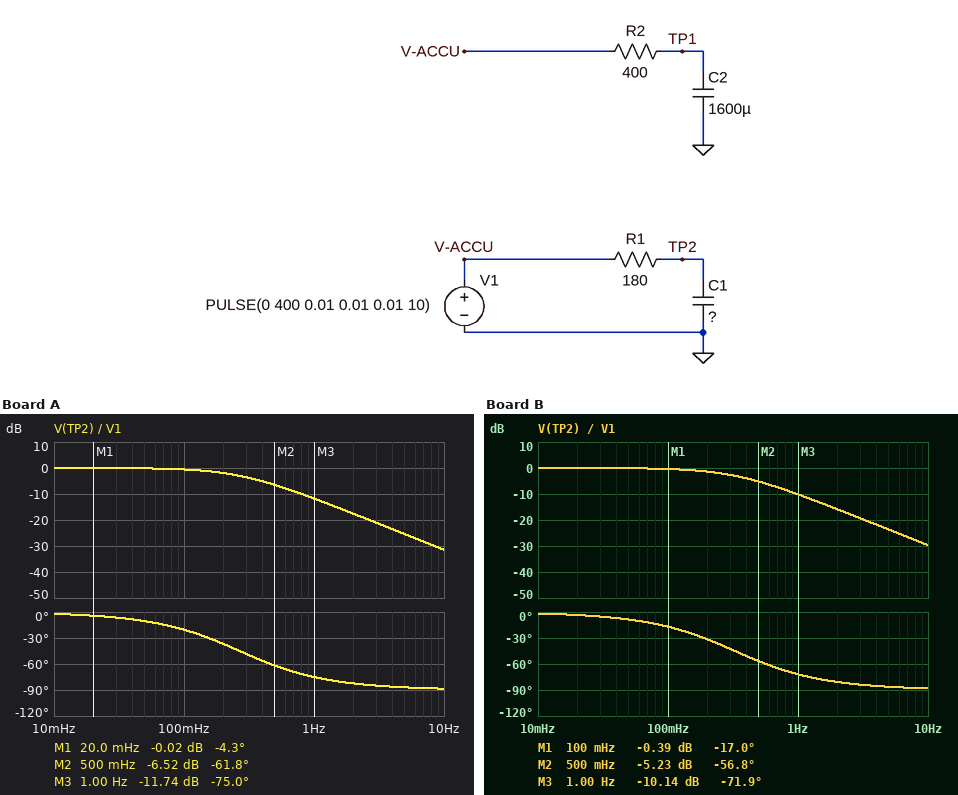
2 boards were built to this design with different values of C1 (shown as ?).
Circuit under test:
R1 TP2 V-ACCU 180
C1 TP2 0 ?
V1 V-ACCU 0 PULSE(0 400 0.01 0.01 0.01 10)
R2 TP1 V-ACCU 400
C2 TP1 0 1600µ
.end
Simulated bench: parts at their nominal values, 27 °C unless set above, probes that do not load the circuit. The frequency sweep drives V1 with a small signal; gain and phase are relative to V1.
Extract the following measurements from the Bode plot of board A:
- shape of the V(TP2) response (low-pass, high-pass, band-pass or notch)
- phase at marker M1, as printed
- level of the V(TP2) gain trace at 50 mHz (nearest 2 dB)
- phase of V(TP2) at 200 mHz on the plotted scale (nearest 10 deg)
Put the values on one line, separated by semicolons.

low-pass; -4.3 deg; 0 dB; -40 deg
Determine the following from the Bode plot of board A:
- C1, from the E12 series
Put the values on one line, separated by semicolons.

3.3 mF
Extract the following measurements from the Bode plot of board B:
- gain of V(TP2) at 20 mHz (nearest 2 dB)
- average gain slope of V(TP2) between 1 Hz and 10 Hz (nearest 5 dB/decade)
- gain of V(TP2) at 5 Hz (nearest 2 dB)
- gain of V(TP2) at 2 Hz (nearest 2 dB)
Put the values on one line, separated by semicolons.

0 dB; -20 dB/decade; -24 dB; -16 dB
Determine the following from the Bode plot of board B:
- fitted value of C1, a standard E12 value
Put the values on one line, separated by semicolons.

2.7 mF
